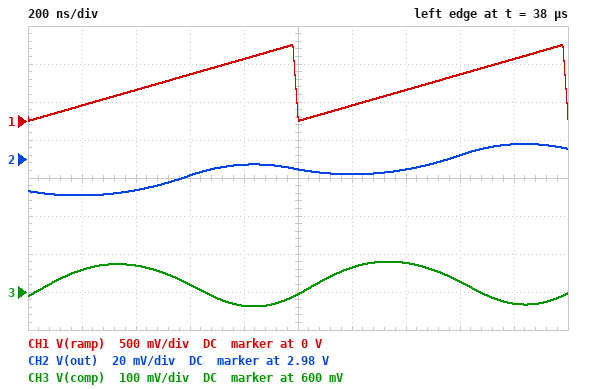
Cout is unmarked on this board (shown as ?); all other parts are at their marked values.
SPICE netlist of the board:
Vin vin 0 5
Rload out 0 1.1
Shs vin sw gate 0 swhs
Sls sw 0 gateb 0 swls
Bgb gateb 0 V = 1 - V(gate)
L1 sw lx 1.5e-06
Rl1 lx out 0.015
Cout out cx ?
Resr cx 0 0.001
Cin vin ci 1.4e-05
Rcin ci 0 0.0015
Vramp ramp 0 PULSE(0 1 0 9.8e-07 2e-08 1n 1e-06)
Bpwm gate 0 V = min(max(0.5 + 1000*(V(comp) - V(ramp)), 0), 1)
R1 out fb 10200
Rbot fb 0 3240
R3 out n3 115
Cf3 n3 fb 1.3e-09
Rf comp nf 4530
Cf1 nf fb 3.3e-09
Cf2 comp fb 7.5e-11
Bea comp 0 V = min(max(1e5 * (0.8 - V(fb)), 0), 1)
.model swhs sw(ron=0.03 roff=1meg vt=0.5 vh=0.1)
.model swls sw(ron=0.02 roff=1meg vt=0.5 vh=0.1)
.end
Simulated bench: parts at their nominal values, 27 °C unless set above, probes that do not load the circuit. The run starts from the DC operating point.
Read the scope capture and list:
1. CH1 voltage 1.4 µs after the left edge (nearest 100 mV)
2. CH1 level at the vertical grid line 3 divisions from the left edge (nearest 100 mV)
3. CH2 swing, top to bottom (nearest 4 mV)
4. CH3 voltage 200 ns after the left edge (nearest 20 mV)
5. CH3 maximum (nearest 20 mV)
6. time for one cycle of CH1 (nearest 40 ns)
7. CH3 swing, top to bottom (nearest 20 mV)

400 mV
600 mV
28 mV
660 mV
680 mV
1.00 µs
120 mV
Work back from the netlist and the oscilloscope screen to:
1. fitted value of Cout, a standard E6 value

10 µF
